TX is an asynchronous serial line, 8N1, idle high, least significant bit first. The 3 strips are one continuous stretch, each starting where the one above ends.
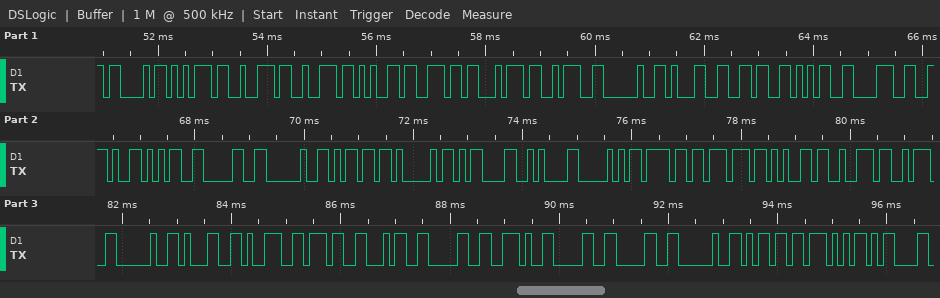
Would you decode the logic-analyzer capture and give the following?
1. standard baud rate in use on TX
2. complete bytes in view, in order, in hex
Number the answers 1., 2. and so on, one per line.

1. 9600 baud
2. 0x43 0x75 0x72 0x72 0x65 0x6E 0x74 0x3A 0x20 0x31 0x36 0x35 0x38 0x2E 0x35 0x30 0x20 0x6D 0x41 0x0D 0x0A 0x50 0x6F 0x77 0x65 0x72 0x3A 0x20 0x31 0x39 0x37 0x34 0x30 0x2E 0x30 0x30 0x20 0x6D 0x57 0x0D
